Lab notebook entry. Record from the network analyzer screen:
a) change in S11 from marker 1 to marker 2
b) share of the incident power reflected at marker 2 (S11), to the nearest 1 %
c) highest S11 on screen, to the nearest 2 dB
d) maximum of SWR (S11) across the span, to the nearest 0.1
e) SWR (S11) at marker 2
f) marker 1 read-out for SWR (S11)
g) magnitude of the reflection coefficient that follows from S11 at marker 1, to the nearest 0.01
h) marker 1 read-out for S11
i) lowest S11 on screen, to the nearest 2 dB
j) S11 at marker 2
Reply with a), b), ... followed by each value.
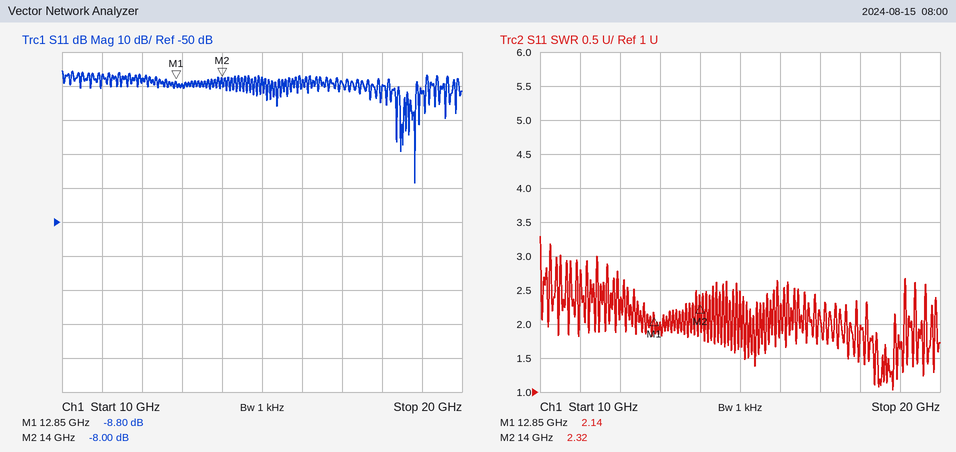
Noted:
a) 0.80 dB
b) 16 %
c) -6 dB
d) 3.3
e) 2.32
f) 2.14
g) 0.36
h) -8.80 dB
i) -38 dB
j) -8.00 dB
